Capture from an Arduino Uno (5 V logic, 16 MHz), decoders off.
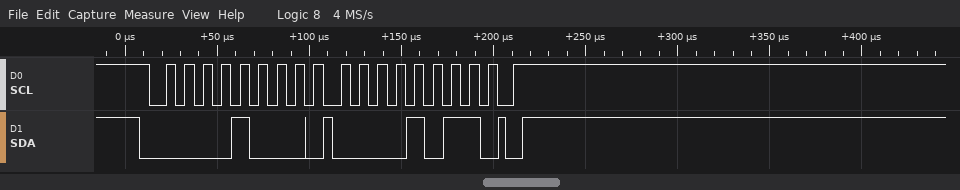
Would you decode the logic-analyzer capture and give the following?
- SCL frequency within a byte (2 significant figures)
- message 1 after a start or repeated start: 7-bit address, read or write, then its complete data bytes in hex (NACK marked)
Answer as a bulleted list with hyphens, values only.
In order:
- 100 kHz
- 0x04 write: 0B
